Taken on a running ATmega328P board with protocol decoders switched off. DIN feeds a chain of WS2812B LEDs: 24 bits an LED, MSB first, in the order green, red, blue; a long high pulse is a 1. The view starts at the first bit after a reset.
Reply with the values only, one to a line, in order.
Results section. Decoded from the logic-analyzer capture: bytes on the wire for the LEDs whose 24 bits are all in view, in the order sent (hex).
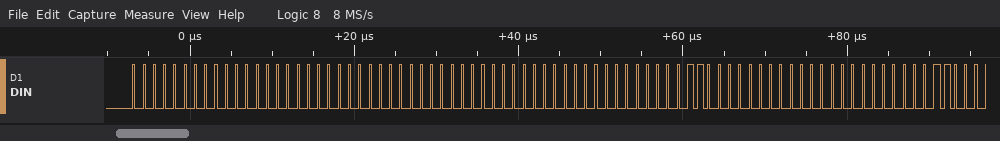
00 00 00 00 00 00 03 00 00
